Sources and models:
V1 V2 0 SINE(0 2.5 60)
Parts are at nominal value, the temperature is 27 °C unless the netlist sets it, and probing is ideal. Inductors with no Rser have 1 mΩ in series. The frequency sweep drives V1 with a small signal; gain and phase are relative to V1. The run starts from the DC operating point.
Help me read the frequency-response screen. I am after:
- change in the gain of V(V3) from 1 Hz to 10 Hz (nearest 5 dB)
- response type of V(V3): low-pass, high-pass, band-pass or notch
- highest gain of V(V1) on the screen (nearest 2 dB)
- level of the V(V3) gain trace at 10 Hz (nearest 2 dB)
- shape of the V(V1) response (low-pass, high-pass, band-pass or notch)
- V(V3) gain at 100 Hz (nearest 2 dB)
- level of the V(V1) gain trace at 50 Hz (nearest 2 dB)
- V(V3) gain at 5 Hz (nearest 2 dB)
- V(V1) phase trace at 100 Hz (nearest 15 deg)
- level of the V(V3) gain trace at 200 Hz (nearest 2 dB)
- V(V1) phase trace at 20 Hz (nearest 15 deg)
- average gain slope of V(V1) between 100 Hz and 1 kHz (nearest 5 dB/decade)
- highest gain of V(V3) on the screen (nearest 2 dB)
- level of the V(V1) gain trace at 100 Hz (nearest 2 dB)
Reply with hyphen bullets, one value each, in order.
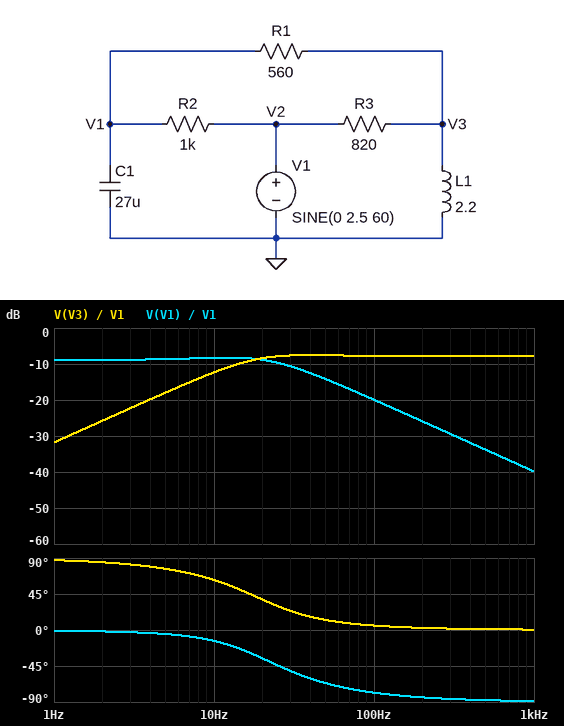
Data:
- 20 dB
- high-pass
- -8 dB
- -12 dB
- low-pass
- -8 dB
- -14 dB
- -18 dB
- -75 deg
- -8 dB
- -30 deg
- -20 dB/decade
- -8 dB
- -20 dB
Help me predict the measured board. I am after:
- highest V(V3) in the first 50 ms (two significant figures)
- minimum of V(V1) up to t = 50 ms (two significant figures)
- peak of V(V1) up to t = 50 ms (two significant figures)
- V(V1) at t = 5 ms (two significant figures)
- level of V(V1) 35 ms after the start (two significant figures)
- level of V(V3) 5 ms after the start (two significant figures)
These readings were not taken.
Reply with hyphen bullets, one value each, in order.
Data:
- 1.0 V
- -420 mV
- 540 mV
- 440 mV
- -240 mV
- 750 mV
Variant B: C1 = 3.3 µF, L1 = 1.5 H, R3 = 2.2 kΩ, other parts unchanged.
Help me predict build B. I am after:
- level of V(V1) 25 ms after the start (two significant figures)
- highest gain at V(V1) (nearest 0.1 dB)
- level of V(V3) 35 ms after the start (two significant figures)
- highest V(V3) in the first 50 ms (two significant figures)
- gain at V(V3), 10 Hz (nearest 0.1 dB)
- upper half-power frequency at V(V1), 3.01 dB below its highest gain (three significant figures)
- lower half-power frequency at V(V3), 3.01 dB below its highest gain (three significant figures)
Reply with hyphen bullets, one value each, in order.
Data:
- 210 mV
- -3.9 dB
- 1.3 V
- 1.4 V
- -19.7 dB
- 143 Hz
- 42.3 Hz
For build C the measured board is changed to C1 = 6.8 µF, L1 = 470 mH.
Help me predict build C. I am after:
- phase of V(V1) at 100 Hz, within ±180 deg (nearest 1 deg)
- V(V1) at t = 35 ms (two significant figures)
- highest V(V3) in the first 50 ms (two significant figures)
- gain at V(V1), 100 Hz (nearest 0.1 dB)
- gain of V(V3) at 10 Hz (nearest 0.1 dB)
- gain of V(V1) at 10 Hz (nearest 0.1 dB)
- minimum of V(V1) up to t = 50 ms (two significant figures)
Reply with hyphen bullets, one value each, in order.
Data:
- -43 deg
- 170 mV
- 710 mV
- -10.2 dB
- -25.2 dB
- -8.9 dB
- -900 mV
